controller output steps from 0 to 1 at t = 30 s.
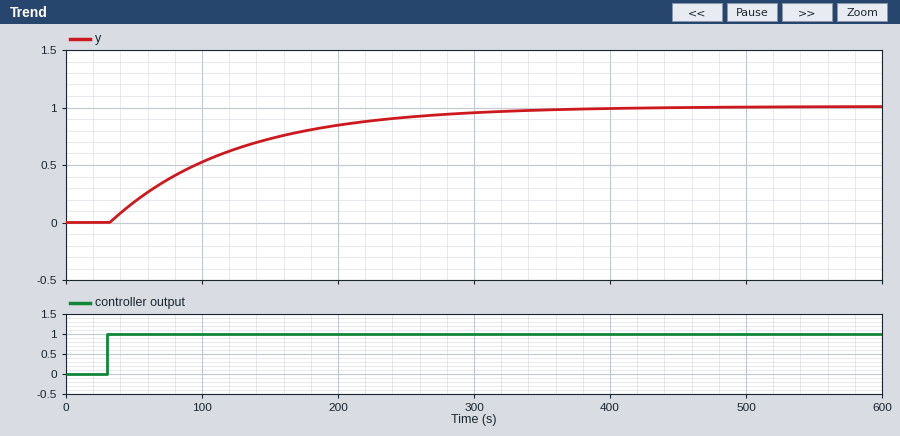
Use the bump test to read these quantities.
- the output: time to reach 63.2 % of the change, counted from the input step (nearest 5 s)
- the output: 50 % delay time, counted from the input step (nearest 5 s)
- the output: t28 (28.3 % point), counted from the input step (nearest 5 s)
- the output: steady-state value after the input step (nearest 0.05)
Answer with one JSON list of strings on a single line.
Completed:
["95 s", "65 s", "35 s", "1.00"]
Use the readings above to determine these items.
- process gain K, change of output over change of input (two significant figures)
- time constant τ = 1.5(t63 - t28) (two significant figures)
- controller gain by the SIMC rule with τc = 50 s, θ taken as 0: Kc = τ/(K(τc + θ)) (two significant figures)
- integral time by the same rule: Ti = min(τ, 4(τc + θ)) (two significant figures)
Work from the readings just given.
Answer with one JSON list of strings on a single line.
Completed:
["1.0", "90 s", "1.8", "90 s"]
